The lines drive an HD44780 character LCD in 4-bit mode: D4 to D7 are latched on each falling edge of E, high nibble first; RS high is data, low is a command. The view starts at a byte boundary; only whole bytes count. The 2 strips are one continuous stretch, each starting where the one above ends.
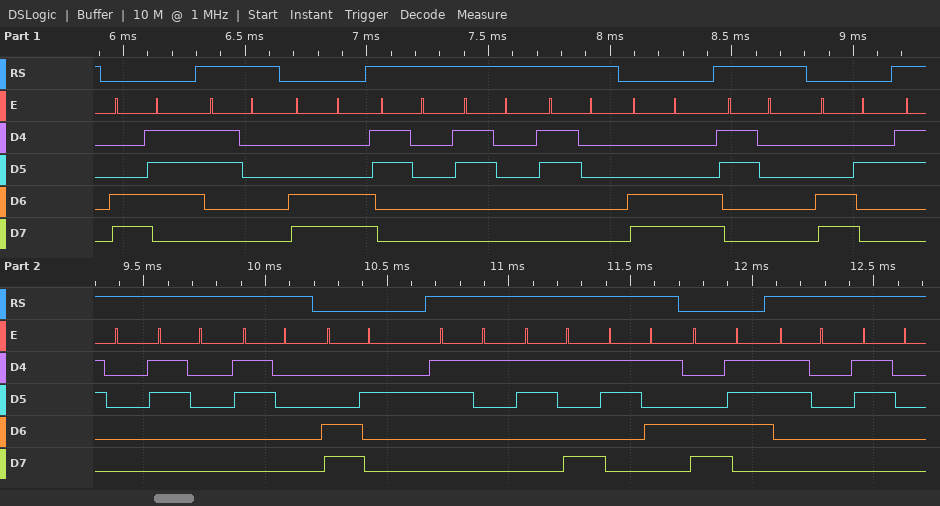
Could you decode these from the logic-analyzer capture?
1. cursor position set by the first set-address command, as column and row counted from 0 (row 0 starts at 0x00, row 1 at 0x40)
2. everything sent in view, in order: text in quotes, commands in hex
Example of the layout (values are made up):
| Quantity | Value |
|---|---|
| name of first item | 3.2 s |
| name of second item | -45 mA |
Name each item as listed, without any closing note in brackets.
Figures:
| Quantity | Value |
|---|---|
| cursor position set by the first set-address command, as column and row counted from 0 | column 7, row 1 |
| everything sent in view, in order: text in quotes, commands in hex | 0xC7 "0" 0xCC "000" 0xCC "0" 0xC2 "000" 0xC2 "195" 0xC7 "00" |
